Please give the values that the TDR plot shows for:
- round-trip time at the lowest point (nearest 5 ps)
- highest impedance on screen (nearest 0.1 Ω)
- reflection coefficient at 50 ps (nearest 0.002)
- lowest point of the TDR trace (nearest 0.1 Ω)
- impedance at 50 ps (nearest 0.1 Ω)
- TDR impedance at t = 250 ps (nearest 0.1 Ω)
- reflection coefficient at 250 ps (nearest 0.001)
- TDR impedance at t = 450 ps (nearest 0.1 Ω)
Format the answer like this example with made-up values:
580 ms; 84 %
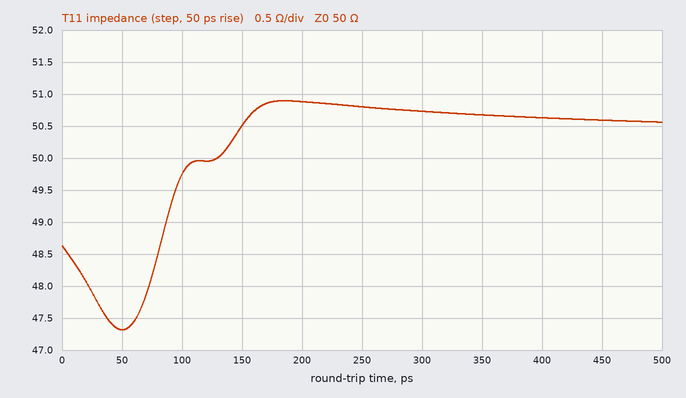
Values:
50 ps; 50.9 Ω; -0.028; 47.3 Ω; 47.3 Ω; 50.8 Ω; +0.008; 50.6 Ω
